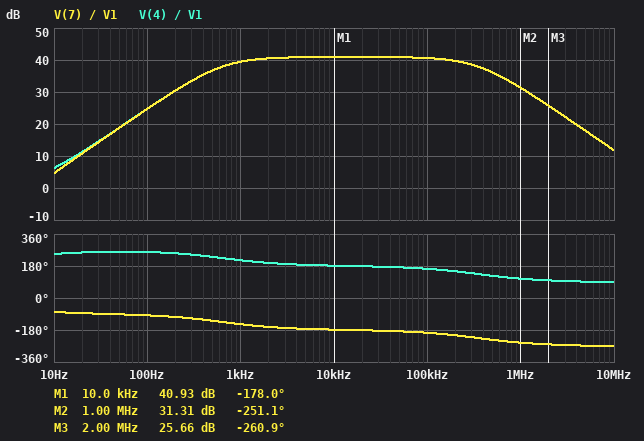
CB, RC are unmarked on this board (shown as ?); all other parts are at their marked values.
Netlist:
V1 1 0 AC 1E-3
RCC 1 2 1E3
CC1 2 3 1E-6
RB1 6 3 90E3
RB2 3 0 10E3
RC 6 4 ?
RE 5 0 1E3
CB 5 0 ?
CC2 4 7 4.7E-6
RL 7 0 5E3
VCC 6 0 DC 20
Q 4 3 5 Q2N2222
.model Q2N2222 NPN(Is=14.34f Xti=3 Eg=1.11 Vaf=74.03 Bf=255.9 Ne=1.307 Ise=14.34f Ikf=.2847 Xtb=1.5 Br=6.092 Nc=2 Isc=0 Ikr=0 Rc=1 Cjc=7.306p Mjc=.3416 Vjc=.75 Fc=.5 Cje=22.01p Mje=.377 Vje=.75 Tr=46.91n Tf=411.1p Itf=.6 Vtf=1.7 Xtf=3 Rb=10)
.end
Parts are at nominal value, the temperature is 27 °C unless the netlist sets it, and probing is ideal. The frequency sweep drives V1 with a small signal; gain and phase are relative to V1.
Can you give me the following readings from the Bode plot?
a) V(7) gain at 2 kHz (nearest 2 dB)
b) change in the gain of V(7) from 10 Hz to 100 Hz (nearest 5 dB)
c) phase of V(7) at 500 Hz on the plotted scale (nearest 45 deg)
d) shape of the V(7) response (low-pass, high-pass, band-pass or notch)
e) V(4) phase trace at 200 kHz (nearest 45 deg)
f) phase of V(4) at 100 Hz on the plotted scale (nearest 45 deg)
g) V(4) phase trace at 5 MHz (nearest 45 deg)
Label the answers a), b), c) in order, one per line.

a) 40 dB
b) 20 dB
c) -135 deg
d) band-pass
e) 135 deg
f) 270 deg
g) 90 deg
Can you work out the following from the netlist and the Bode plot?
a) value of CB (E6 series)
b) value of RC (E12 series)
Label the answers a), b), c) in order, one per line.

a) 10 µF
b) 10 kΩ
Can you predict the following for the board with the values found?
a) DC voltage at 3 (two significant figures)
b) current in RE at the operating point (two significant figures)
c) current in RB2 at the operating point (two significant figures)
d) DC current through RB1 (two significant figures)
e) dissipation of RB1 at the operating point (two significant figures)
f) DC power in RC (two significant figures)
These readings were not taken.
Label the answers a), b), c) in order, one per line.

a) 1.9 V
b) 1.3 mA
c) 190 µA
d) 200 µA
e) 3.6 mW
f) 16 mW
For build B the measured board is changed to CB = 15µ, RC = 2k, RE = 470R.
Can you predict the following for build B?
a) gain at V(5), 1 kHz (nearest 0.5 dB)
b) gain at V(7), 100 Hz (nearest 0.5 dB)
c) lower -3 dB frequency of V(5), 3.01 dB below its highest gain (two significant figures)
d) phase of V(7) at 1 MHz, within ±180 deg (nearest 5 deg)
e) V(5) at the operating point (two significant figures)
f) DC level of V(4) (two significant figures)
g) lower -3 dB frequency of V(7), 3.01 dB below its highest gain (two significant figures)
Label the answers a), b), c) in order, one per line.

a) -6.0 dB
b) 21.0 dB
c) 16 Hz
d) 120 deg
e) 1.2 V
f) 15 V
g) 760 Hz
